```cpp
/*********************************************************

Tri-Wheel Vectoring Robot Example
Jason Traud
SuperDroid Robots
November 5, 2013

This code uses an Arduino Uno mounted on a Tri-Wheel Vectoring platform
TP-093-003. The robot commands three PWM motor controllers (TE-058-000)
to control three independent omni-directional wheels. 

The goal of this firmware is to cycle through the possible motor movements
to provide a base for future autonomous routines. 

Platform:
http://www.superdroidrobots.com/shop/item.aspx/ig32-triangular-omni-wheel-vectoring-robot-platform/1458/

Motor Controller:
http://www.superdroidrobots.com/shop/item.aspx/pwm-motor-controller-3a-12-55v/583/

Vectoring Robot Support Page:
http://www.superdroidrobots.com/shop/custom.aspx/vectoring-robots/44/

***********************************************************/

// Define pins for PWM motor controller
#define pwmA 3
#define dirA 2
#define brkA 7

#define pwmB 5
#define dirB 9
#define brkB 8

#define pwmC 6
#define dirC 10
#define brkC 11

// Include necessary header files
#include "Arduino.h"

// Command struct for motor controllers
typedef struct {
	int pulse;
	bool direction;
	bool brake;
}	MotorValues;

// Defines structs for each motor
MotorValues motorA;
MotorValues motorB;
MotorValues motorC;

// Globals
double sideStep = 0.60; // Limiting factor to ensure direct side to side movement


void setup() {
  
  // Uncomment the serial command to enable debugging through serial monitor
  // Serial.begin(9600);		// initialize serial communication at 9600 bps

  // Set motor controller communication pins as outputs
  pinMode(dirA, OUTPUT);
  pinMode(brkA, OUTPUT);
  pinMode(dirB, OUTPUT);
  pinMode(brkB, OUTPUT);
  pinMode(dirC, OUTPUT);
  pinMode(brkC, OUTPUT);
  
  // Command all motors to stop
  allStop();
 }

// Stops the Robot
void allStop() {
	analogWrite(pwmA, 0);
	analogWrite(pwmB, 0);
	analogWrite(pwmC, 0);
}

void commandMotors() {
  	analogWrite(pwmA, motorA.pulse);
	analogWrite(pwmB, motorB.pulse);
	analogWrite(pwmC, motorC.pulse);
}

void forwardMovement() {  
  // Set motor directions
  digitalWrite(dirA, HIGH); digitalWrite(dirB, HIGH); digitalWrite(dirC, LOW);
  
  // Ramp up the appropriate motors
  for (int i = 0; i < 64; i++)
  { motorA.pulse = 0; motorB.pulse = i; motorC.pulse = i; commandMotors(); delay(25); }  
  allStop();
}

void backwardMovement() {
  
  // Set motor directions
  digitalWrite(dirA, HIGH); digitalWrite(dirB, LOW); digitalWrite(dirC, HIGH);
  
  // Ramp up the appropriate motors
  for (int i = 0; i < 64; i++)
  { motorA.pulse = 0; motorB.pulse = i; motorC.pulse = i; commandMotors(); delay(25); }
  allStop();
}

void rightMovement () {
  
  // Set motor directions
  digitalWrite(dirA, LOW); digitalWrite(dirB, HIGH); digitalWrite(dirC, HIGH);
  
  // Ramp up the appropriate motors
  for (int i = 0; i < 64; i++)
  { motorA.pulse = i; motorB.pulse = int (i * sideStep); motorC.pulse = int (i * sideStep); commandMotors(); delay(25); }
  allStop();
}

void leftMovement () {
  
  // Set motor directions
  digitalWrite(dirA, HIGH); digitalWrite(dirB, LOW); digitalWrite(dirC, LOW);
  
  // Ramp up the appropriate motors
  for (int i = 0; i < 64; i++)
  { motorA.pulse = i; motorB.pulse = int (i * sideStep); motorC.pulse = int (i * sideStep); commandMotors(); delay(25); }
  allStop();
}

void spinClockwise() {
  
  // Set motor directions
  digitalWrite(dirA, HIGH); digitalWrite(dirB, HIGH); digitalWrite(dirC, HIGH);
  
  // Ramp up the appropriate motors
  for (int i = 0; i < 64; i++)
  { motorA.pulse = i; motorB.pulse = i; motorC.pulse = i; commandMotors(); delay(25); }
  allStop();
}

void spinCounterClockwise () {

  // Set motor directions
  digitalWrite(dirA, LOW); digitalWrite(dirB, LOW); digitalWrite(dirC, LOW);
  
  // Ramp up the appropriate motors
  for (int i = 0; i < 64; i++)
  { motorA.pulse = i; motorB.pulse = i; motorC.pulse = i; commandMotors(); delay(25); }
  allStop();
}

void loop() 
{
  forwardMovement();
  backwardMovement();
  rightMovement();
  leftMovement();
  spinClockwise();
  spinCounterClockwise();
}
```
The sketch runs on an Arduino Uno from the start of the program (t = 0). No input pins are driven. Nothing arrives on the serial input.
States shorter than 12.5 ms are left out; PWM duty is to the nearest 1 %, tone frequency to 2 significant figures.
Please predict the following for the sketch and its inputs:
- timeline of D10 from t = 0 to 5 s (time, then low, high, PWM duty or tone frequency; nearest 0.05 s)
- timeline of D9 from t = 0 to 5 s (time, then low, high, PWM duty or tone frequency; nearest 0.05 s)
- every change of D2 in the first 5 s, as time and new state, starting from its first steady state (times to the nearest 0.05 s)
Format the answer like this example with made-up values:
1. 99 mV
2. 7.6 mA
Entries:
1. 0 s low; 1.6 s high; 4.8 s low
2. 0 s high; 1.6 s low; 3.2 s high; 4.8 s low
3. 0 s high; 3.2 s low; 4.8 s high
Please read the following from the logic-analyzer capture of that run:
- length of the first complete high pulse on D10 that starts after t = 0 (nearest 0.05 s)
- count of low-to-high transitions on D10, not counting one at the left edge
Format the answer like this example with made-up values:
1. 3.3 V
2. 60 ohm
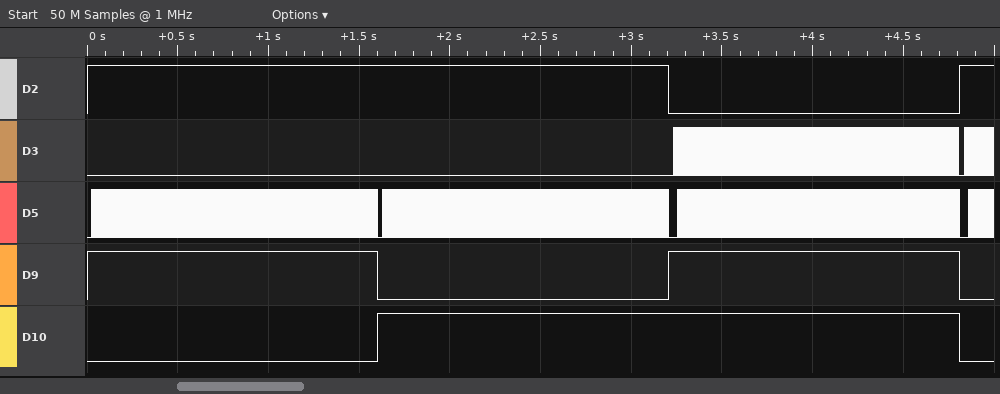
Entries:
1. 3.20 s
2. 1
